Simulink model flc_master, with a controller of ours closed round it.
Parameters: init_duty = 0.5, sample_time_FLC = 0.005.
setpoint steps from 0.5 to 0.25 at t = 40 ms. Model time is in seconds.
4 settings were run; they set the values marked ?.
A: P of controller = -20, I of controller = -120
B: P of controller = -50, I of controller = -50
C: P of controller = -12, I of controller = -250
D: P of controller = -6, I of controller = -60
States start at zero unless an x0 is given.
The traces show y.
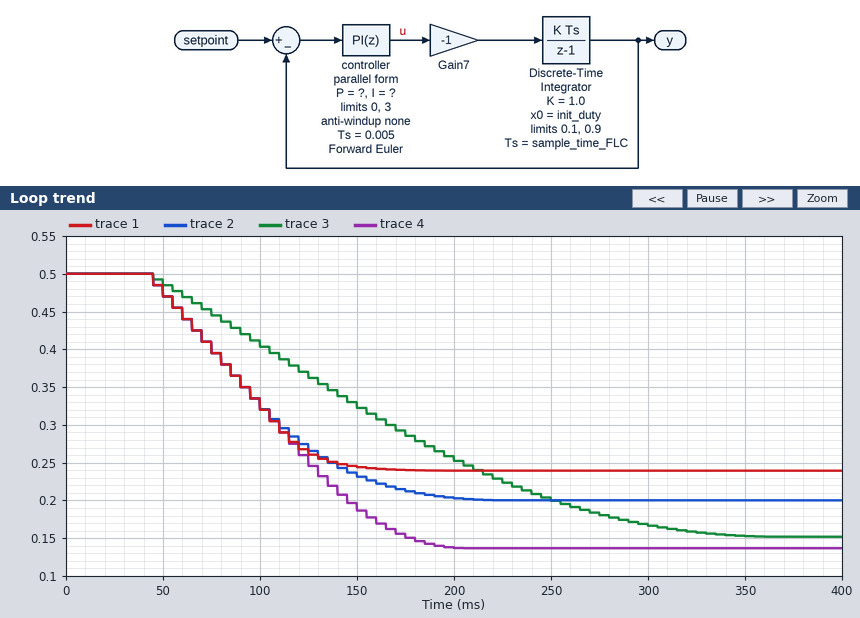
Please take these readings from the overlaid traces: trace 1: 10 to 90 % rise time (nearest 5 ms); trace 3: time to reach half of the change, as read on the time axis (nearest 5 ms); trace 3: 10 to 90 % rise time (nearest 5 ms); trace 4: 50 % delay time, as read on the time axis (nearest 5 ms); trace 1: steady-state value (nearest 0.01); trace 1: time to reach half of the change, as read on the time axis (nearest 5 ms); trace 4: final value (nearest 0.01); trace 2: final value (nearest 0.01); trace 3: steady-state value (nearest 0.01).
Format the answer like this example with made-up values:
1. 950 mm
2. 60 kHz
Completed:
1. 75 ms
2. 150 ms
3. 205 ms
4. 105 ms
5. 0.24
6. 85 ms
7. 0.14
8. 0.20
9. 0.15
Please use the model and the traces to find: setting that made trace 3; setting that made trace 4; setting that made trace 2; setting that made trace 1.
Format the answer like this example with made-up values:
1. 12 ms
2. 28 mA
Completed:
1. D
2. C
3. A
4. B
